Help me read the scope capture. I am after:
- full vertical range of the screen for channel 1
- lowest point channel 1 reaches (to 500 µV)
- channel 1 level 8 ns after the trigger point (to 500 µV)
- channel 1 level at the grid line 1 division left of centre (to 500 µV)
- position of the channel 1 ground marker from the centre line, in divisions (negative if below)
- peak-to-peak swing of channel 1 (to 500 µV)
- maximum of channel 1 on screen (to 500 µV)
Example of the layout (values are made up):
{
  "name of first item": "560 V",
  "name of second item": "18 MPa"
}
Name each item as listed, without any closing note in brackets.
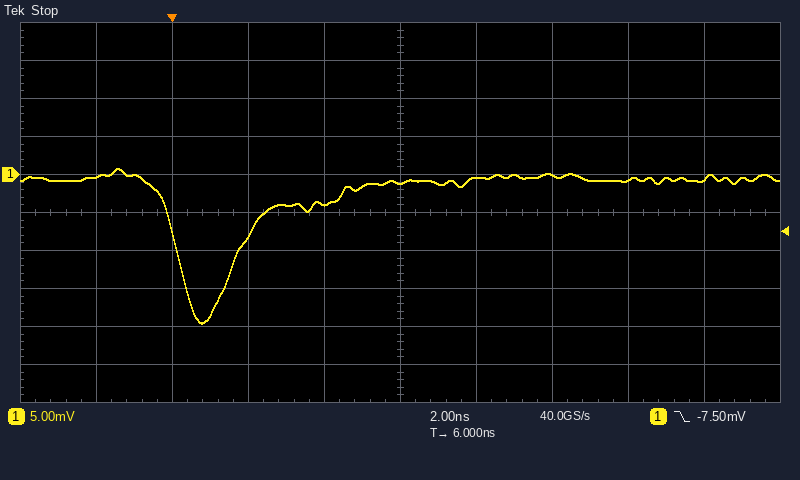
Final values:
{
  "full vertical range of the screen for channel 1": "50 mV",
  "lowest point channel 1 reaches": "-19.5 mV",
  "channel 1 level 8 ns after the trigger point": "-500 µV",
  "channel 1 level at the grid line 1 division left of centre": "-4.0 mV",
  "position of the channel 1 ground marker from the centre line, in divisions": "+1.0 div",
  "peak-to-peak swing of channel 1": "20.5 mV",
  "maximum of channel 1 on screen": "1.0 mV"
}
